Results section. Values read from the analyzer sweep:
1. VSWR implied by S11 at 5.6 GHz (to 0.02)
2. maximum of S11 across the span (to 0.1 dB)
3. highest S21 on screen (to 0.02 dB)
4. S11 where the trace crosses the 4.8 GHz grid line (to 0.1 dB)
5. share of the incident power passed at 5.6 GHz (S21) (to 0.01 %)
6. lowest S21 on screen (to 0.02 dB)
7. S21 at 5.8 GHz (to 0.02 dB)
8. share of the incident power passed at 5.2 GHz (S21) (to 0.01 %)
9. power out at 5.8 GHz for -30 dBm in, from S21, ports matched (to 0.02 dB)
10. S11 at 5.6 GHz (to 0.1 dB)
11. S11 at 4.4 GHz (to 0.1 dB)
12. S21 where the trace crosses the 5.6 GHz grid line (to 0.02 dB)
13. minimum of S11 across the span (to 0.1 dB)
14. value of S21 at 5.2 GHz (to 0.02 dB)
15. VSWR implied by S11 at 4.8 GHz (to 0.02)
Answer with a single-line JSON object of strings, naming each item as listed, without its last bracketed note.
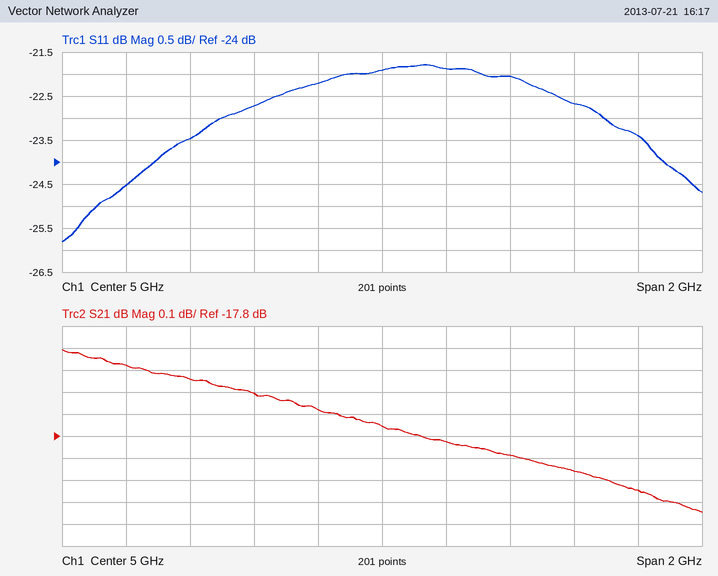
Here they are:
{"VSWR implied by S11 at 5.6 GHz": "1.16", "maximum of S11 across the span": "-21.8 dB", "highest S21 on screen": "-17.40 dB", "S11 where the trace crosses the 4.8 GHz grid line": "-22.2 dB", "share of the incident power passed at 5.6 GHz (S21)": "1.60 %", "lowest S21 on screen": "-18.14 dB", "S21 at 5.8 GHz": "-18.04 dB", "share of the incident power passed at 5.2 GHz (S21)": "1.65 %", "power out at 5.8 GHz for -30 dBm in, from S21, ports matched": "-48.04 dBm", "S11 at 5.6 GHz": "-22.7 dB", "S11 at 4.4 GHz": "-23.5 dB", "S21 where the trace crosses the 5.6 GHz grid line": "-17.96 dB", "minimum of S11 across the span": "-25.8 dB", "value of S21 at 5.2 GHz": "-17.82 dB", "VSWR implied by S11 at 4.8 GHz": "1.16"}
